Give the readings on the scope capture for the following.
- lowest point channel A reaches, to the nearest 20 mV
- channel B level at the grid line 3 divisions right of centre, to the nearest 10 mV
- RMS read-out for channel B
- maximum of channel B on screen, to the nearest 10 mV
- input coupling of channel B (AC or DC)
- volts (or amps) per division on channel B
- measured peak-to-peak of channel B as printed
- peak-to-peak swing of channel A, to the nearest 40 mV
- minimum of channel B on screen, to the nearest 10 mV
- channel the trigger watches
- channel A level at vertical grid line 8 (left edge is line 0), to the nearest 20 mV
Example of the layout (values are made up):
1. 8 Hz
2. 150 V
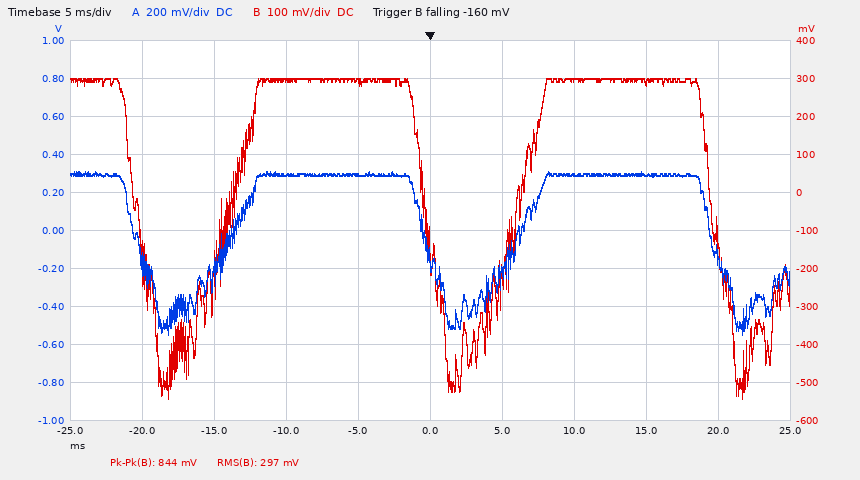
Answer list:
1. -540 mV
2. 290 mV
3. 297 mV
4. 300 mV
5. DC
6. 100 mV
7. 844 mV
8. 840 mV
9. -540 mV
10. channel B
11. 300 mV
